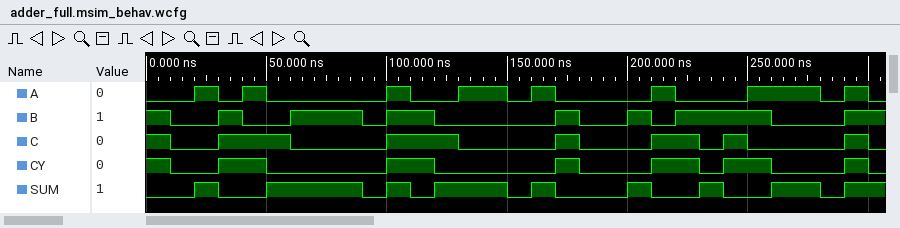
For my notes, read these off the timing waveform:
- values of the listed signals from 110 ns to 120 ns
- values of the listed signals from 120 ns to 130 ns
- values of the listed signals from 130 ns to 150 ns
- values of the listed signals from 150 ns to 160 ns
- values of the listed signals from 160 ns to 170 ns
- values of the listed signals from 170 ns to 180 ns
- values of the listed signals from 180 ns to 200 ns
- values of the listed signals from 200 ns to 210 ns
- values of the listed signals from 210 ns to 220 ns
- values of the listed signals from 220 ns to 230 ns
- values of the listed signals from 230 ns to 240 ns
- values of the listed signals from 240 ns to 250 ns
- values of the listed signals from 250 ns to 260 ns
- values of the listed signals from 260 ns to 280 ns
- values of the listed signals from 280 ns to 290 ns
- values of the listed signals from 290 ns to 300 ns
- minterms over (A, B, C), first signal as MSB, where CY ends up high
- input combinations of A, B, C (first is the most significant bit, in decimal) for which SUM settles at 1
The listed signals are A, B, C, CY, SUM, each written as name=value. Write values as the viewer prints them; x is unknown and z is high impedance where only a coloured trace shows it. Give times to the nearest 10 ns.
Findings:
A=0, B=1, C=1, CY=1, SUM=0
A=0, B=0, C=1, CY=0, SUM=1
A=1, B=0, C=0, CY=0, SUM=1
A=0, B=0, C=0, CY=0, SUM=0
A=1, B=0, C=0, CY=0, SUM=1
A=0, B=1, C=1, CY=1, SUM=0
A=0, B=0, C=0, CY=0, SUM=0
A=0, B=1, C=0, CY=0, SUM=1
A=1, B=0, C=1, CY=1, SUM=0
A=0, B=1, C=1, CY=1, SUM=0
A=0, B=1, C=0, CY=0, SUM=1
A=0, B=1, C=1, CY=1, SUM=0
A=1, B=1, C=0, CY=1, SUM=0
A=1, B=0, C=0, CY=0, SUM=1
A=0, B=0, C=0, CY=0, SUM=0
A=1, B=1, C=1, CY=1, SUM=1
3, 5, 6, 7
1, 2, 4, 7
